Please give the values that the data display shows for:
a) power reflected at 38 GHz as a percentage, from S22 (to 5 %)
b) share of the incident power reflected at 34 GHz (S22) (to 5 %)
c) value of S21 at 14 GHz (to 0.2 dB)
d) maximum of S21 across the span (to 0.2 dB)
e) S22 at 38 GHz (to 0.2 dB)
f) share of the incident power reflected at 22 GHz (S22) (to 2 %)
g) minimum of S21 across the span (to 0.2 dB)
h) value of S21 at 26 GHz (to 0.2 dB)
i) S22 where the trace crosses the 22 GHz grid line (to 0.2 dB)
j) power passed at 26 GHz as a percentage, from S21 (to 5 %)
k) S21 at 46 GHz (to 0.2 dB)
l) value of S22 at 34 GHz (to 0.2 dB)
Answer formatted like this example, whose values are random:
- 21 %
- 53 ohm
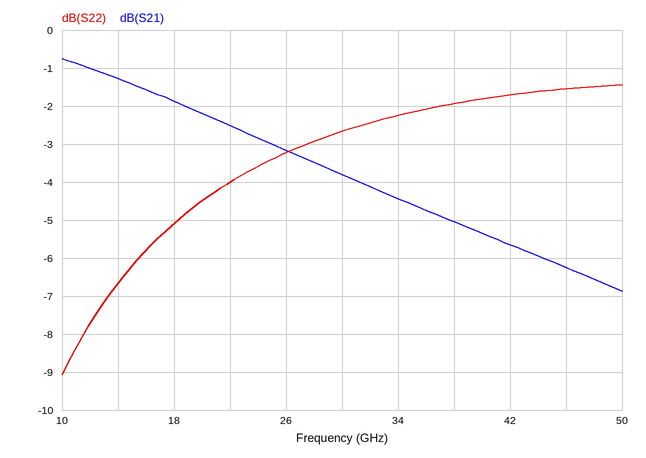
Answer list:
- 65 %
- 60 %
- -1.2 dB
- -0.8 dB
- -2.0 dB
- 40 %
- -6.8 dB
- -3.2 dB
- -4.0 dB
- 50 %
- -6.2 dB
- -2.2 dB
